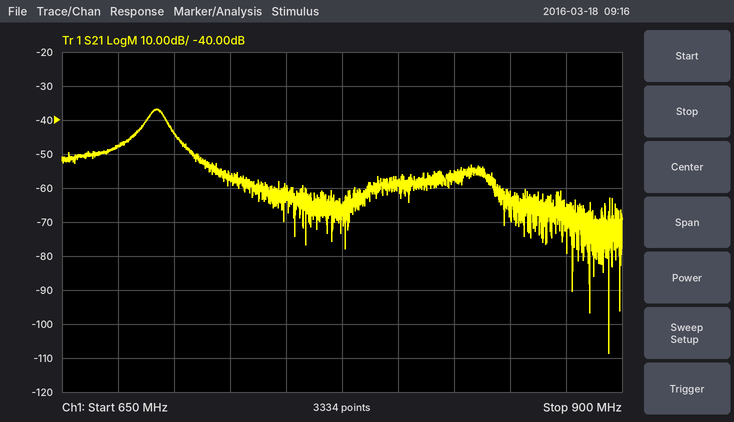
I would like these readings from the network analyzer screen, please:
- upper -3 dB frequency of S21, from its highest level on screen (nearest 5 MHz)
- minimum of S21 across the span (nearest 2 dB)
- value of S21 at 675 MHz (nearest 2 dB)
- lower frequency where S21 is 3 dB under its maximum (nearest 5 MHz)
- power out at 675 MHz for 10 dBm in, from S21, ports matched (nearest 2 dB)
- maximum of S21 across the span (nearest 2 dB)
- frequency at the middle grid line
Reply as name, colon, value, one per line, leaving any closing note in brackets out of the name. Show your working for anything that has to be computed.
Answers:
upper -3 dB frequency of S21, from its highest level on screen: 695 MHz
minimum of S21 across the span: -108 dB
value of S21 at 675 MHz: -48 dB
lower frequency where S21 is 3 dB under its maximum: 690 MHz
power out at 675 MHz for 10 dBm in, from S21, ports matched: 10 dBm + (-48 dB) = -38 dBm
maximum of S21 across the span: -36 dB
frequency at the middle grid line: 775 MHz
